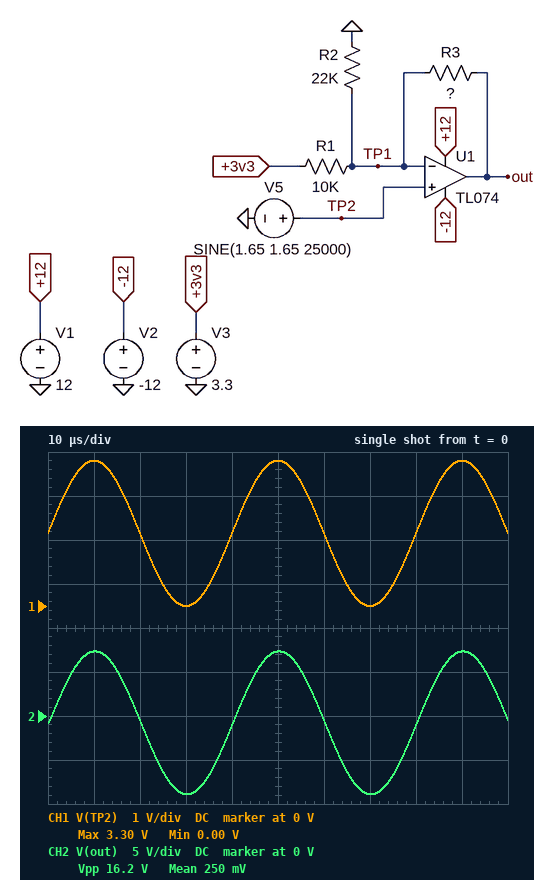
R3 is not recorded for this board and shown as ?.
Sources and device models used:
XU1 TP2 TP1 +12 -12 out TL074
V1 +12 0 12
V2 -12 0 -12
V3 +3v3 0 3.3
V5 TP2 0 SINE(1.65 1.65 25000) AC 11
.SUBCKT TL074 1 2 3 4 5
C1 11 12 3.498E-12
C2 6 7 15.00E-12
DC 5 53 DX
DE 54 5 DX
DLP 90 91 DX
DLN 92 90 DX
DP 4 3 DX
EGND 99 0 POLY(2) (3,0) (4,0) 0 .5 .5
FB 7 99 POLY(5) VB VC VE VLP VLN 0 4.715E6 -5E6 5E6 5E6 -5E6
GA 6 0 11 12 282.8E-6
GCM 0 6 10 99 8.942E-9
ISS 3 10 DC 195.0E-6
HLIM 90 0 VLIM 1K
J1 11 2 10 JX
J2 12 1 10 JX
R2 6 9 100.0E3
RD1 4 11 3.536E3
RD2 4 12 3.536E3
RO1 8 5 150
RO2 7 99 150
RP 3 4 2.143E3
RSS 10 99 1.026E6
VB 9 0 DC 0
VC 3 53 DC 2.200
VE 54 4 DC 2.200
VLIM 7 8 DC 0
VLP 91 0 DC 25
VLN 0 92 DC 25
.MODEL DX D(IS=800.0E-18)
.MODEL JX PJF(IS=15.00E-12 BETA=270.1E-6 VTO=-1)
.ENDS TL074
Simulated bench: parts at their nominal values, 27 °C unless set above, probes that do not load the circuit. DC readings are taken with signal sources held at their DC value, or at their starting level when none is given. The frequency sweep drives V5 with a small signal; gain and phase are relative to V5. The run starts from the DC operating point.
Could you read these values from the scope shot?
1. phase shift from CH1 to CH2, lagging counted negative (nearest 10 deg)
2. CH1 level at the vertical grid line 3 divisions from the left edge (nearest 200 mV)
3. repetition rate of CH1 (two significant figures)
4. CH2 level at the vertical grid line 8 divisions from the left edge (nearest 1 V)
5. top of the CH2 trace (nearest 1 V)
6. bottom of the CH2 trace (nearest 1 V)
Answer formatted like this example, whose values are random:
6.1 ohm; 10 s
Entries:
0 deg; 0 V; 25 kHz; -1 V; 7 V; -9 V
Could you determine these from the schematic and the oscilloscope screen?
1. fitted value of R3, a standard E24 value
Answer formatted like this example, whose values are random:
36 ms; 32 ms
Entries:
27 kΩ
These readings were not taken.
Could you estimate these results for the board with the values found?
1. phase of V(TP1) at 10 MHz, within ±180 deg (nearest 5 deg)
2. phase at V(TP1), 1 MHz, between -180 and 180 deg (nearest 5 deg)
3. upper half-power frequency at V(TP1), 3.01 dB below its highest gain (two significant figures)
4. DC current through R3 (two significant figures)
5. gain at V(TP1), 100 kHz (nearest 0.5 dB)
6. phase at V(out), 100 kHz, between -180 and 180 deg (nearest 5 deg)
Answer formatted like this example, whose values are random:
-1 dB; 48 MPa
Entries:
-145 deg; -60 deg; 780 kHz; 90 µA; 0 dB; -10 deg
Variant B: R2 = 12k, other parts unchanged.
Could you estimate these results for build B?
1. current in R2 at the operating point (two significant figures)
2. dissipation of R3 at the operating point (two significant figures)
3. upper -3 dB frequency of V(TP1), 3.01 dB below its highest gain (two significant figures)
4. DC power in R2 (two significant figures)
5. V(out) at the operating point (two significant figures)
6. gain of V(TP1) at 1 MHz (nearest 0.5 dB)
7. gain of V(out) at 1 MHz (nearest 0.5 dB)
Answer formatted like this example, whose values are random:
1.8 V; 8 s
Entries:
140 µA; 20 µW; 630 kHz; 230 µW; 910 mV; -5.5 dB; 10.0 dB
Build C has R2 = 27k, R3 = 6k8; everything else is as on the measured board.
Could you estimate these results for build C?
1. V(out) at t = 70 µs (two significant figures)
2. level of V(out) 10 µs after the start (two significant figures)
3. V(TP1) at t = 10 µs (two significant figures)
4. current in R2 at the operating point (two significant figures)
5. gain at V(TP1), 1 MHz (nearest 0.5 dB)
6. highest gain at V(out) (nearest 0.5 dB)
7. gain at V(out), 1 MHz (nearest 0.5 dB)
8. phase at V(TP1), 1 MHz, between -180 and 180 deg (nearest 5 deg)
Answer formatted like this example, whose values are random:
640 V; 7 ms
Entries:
-2.2 V; 4.1 V; 3.3 V; 61 µA; -0.5 dB; 5.5 dB; 5.0 dB; -30 deg
